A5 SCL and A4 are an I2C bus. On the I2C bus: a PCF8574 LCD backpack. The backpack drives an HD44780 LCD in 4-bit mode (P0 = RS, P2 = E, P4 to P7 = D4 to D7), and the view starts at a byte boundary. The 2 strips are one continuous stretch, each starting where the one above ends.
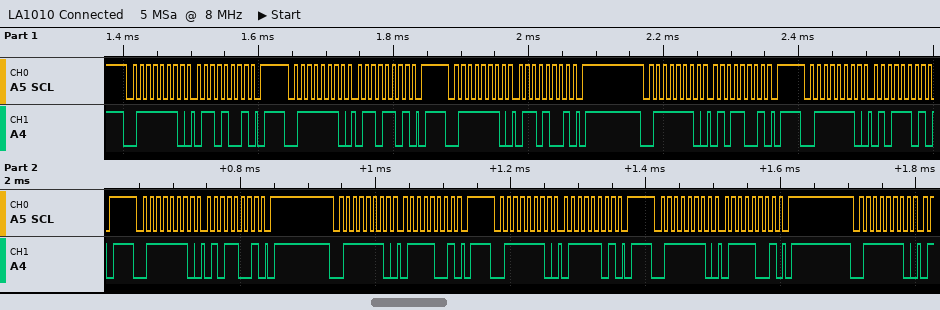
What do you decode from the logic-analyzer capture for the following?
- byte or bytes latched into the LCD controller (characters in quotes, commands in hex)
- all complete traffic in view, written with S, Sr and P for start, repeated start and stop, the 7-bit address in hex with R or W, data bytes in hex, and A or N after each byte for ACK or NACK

'e'
S 3FW A 69 A P S 3FW A 6D A P S 3FW A 69 A P S 3FW A 59 A P S 3FW A 5D A P S 3FW A 59 A P S 3FW A 79 A P S 3FW A 7D A P S 3FW A 79 A P S 3FW A
